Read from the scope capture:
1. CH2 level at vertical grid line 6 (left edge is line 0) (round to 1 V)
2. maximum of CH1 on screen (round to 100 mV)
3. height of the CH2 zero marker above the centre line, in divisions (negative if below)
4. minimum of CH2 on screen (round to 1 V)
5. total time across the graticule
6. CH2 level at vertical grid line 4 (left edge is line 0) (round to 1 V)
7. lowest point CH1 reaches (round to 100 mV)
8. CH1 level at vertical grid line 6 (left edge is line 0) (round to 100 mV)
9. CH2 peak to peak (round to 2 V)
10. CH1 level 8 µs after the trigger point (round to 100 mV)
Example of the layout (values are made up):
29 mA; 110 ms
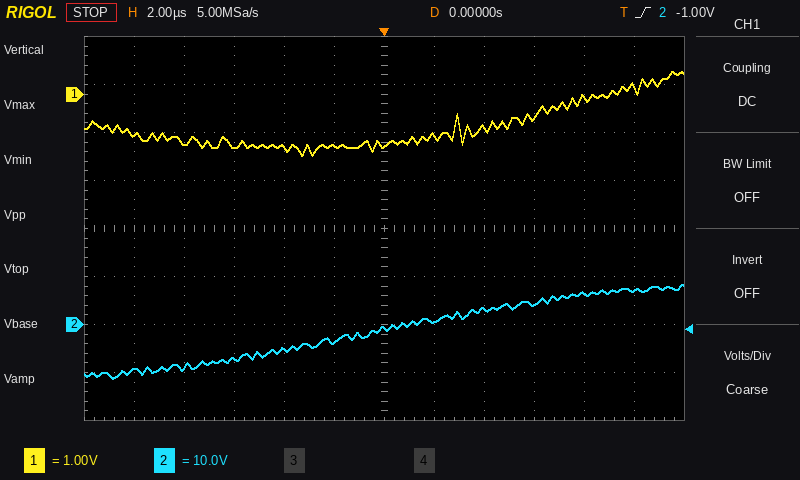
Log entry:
-1 V; 500 mV; -2.0 div; -11 V; 24 µs; -5 V; -1.3 V; -1.1 V; 20 V; -100 mV
